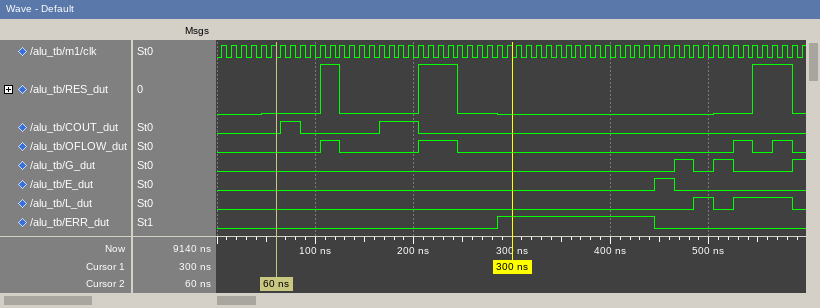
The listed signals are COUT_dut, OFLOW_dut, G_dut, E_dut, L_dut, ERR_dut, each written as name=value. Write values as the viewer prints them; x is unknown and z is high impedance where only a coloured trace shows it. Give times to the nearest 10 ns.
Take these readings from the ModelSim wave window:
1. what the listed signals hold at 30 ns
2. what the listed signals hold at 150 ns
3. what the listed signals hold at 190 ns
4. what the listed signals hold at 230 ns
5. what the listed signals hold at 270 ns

COUT_dut=0, OFLOW_dut=0, G_dut=0, E_dut=0, L_dut=0, ERR_dut=0
COUT_dut=0, OFLOW_dut=0, G_dut=0, E_dut=0, L_dut=0, ERR_dut=0
COUT_dut=1, OFLOW_dut=0, G_dut=0, E_dut=0, L_dut=0, ERR_dut=0
COUT_dut=0, OFLOW_dut=1, G_dut=0, E_dut=0, L_dut=0, ERR_dut=0
COUT_dut=0, OFLOW_dut=0, G_dut=0, E_dut=0, L_dut=0, ERR_dut=0
